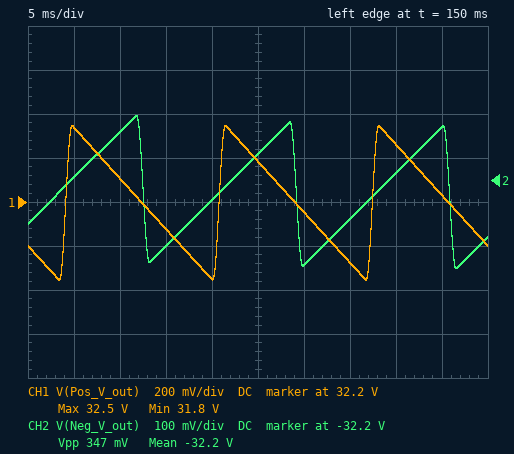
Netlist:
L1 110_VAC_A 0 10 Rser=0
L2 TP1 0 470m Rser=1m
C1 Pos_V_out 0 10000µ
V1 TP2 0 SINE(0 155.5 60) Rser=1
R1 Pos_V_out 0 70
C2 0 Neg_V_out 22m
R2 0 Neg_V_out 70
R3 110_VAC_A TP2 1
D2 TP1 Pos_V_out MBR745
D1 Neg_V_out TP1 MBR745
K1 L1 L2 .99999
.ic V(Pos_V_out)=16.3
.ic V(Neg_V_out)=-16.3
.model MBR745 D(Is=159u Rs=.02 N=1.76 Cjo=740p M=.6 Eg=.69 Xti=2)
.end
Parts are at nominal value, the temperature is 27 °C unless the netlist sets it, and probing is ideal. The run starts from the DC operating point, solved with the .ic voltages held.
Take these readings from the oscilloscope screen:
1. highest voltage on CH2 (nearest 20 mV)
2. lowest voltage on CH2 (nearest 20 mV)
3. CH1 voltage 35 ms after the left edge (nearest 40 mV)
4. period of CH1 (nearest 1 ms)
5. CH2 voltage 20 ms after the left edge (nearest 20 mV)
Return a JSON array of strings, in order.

["-32.06 V", "-32.40 V", "31.92 V", "17 ms", "-32.24 V"]
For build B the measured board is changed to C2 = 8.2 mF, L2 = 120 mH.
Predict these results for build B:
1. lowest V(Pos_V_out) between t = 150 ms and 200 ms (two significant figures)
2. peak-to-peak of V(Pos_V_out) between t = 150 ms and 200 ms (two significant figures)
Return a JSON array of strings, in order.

["16 V", "360 mV"]
